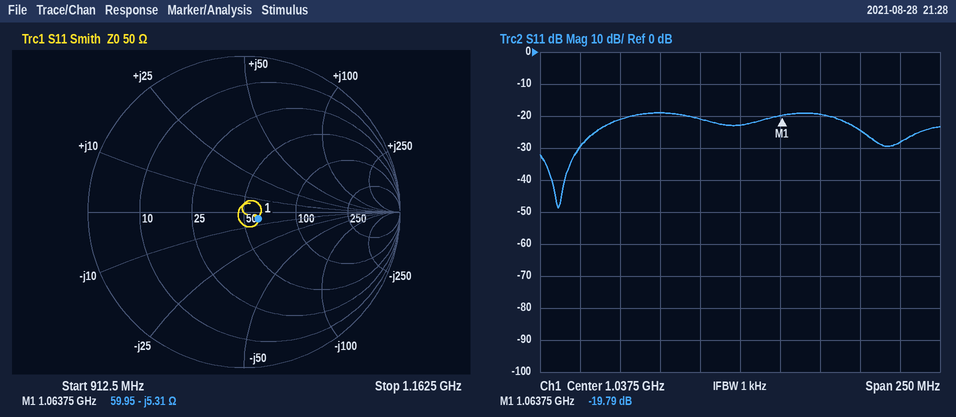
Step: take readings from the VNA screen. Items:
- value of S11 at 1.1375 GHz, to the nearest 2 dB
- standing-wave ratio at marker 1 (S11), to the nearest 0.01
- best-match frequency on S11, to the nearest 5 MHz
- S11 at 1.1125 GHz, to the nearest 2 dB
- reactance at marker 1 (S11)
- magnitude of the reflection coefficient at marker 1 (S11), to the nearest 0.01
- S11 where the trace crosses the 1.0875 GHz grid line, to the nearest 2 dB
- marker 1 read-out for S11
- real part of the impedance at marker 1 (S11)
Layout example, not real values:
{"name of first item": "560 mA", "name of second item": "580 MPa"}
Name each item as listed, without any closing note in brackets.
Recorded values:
{"value of S11 at 1.1375 GHz, to the nearest 2 dB": "-28 dB", "standing-wave ratio at marker 1 (S11), to the nearest 0.01": "1.23", "best-match frequency on S11, to the nearest 5 MHz": "925 MHz", "S11 at 1.1125 GHz, to the nearest 2 dB": "-24 dB", "reactance at marker 1": "-5.31 Ω", "magnitude of the reflection coefficient at marker 1 (S11), to the nearest 0.01": "0.10", "S11 where the trace crosses the 1.0875 GHz grid line, to the nearest 2 dB": "-20 dB", "marker 1 read-out for S11": "-19.79 dB", "real part of the impedance at marker 1": "59.95 Ω"}
